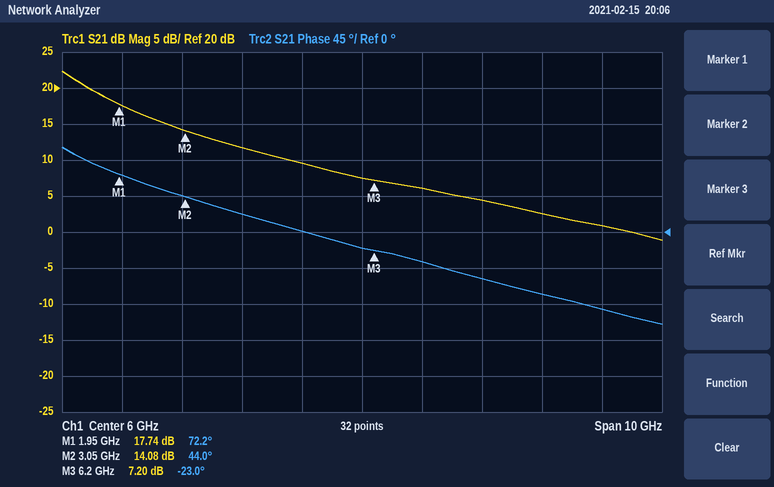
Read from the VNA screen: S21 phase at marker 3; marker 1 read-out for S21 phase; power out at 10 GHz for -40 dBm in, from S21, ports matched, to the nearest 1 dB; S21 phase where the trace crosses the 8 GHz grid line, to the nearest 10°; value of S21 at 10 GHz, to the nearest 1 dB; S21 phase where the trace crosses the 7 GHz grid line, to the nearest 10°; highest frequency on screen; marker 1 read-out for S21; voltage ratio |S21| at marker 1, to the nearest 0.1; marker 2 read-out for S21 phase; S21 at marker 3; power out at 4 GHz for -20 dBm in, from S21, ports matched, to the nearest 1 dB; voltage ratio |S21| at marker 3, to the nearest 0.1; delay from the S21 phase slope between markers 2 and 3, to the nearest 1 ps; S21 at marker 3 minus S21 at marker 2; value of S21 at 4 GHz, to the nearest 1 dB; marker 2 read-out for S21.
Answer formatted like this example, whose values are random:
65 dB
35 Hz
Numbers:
-23.0°
72.2°
-39 dBm
-60°
1 dB
-40°
11 GHz
17.74 dB
7.7
44.0°
7.20 dB
-8 dBm
2.3
59 ps
-6.88 dB
12 dB
14.08 dB
